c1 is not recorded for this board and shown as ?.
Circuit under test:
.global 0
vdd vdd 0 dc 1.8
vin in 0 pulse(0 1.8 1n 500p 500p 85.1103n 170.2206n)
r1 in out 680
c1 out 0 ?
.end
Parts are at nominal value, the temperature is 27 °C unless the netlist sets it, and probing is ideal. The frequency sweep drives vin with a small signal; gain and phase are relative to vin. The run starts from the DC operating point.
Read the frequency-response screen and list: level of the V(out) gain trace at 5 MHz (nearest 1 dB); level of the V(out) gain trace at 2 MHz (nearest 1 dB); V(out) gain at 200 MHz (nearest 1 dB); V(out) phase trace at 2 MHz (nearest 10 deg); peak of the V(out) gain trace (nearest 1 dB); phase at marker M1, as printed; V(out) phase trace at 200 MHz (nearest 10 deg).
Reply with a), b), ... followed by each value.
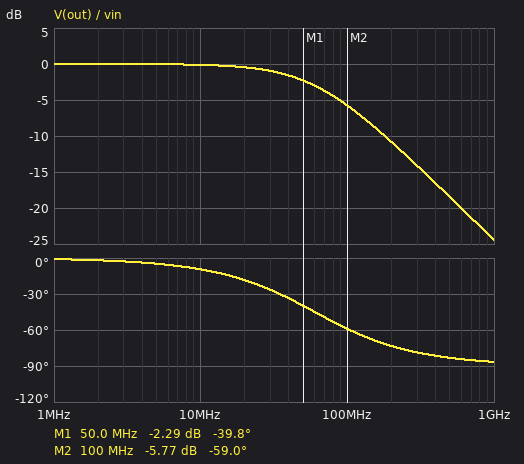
a) 0 dB
b) 0 dB
c) -11 dB
d) 0 deg
e) 0 dB
f) -39.8 deg
g) -70 deg
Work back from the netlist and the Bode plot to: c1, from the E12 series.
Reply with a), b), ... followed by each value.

a) 3.9 pF
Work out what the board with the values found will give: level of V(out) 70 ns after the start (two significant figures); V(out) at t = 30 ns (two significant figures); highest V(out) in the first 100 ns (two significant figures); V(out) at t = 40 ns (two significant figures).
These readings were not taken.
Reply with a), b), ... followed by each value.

a) 1.8 V
b) 1.8 V
c) 1.8 V
d) 1.8 V
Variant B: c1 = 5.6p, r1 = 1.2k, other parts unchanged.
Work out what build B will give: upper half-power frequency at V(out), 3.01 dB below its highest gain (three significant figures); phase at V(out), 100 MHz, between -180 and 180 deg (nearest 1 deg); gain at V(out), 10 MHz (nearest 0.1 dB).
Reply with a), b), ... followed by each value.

a) 23.7 MHz
b) -77 deg
c) -0.7 dB
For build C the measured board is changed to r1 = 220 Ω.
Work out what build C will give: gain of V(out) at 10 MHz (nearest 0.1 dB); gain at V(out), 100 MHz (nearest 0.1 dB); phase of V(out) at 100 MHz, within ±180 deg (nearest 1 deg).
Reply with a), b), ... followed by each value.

a) 0 dB
b) -1.1 dB
c) -28 deg
